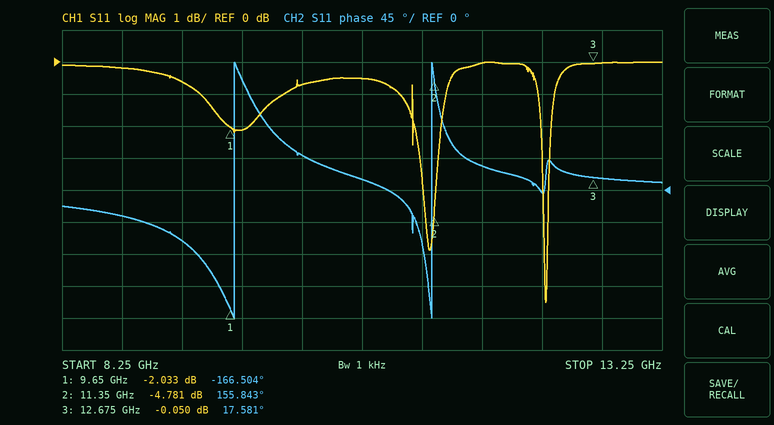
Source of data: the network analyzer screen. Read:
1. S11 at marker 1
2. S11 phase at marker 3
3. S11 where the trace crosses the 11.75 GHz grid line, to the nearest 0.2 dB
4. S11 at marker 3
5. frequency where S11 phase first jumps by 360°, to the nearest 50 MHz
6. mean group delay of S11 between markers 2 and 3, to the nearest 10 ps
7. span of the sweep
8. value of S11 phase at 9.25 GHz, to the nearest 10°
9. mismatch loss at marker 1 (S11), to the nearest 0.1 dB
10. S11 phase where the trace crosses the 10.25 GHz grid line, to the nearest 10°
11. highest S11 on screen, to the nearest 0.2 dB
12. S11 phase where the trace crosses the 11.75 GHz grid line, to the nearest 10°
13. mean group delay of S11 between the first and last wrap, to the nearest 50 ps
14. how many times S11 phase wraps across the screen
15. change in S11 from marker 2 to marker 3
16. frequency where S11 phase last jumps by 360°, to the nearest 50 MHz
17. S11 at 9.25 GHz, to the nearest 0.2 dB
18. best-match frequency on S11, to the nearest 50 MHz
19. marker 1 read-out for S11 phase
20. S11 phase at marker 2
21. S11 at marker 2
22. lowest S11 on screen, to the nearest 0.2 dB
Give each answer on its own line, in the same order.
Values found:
-2.033 dB
17.581°
0.0 dB
-0.050 dB
9.70 GHz
290 ps
5 GHz
-70°
4.3 dB
50°
0.0 dB
30°
600 ps
2
4.731 dB
11.35 GHz
-0.6 dB
12.30 GHz
-166.504°
155.843°
-4.781 dB
-7.6 dB
